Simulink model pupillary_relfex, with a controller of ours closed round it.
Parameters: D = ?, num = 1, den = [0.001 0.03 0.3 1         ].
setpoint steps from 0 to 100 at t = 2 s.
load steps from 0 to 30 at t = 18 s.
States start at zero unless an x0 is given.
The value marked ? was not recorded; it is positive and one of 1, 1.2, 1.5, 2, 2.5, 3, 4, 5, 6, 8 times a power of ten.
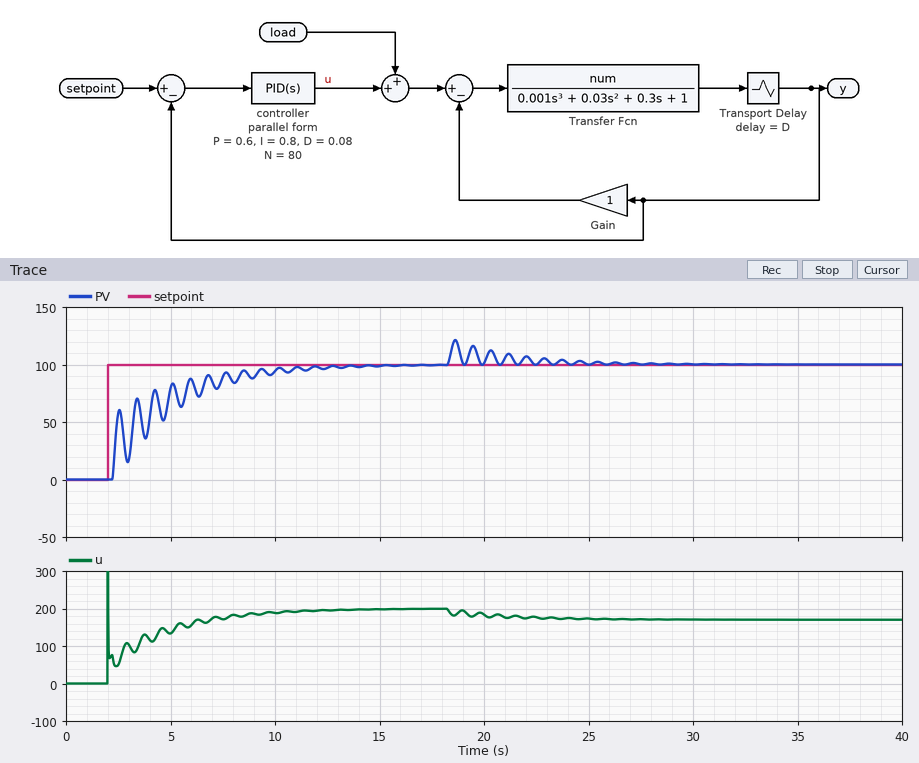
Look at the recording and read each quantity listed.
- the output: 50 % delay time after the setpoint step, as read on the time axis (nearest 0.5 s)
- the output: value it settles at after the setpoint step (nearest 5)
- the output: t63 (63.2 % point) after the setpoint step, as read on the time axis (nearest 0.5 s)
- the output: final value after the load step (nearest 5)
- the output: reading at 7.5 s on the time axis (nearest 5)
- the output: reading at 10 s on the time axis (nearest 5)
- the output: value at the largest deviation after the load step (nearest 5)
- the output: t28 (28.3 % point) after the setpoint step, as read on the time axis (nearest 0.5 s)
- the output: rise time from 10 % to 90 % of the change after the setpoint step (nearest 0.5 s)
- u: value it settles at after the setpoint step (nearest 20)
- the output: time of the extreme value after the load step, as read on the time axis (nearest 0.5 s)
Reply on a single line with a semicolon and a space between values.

2.5 s; 100; 3.5 s; 100; 90; 95; 120; 2.5 s; 4.5 s; 200; 18.5 s
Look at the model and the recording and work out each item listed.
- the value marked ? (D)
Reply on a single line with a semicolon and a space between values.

0.2
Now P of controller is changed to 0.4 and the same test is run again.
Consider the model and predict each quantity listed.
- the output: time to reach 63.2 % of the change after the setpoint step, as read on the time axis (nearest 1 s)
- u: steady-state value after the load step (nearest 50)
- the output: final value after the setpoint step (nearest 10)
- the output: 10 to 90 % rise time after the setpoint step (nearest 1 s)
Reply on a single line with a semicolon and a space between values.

4 s; 150; 100; 6 s
